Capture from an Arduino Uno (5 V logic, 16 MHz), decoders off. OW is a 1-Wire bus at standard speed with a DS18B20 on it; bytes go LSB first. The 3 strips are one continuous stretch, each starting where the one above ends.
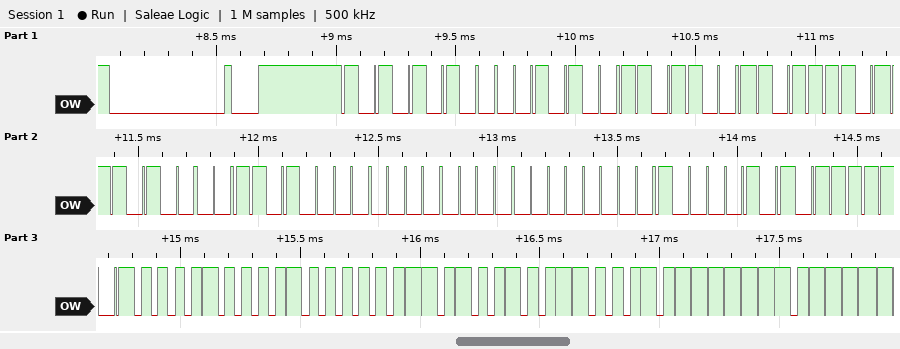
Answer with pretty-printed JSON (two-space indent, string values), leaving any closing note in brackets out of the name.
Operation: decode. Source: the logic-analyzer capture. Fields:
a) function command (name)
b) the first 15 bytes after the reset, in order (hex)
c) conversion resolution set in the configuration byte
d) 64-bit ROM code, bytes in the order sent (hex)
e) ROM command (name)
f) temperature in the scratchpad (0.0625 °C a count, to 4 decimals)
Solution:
{
  "function command": "Read Scratchpad",
  "the first 15 bytes after the reset, in order": "55 28 9B BD 0B 0B 00 00 A1 BE 10 02 4B 46 7F",
  "conversion resolution set in the configuration byte": "12 bits",
  "64-bit ROM code, bytes in the order sent": "28 9B BD 0B 0B 00 00 A1",
  "ROM command": "Match ROM",
  "temperature in the scratchpad": "33.0000 °C"
}
